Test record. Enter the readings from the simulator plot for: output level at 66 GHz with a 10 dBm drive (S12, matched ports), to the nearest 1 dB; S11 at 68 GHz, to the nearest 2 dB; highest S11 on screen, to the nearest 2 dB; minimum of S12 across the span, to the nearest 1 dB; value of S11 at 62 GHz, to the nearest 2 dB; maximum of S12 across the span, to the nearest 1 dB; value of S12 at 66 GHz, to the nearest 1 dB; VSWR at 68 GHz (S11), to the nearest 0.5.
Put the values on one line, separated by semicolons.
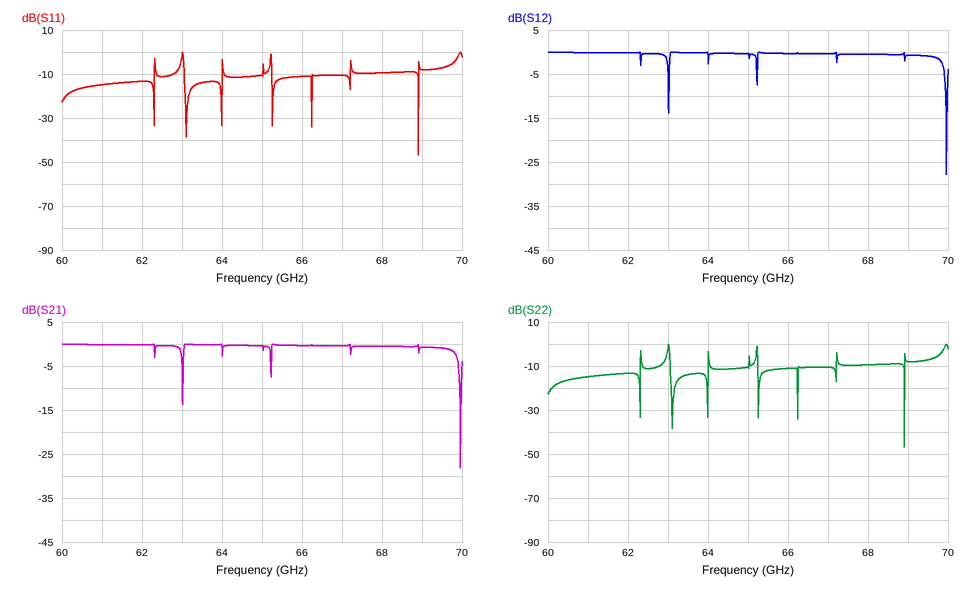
10 dBm; -10 dB; 0 dB; -28 dB; -14 dB; 0 dB; 0 dB; 2.0
